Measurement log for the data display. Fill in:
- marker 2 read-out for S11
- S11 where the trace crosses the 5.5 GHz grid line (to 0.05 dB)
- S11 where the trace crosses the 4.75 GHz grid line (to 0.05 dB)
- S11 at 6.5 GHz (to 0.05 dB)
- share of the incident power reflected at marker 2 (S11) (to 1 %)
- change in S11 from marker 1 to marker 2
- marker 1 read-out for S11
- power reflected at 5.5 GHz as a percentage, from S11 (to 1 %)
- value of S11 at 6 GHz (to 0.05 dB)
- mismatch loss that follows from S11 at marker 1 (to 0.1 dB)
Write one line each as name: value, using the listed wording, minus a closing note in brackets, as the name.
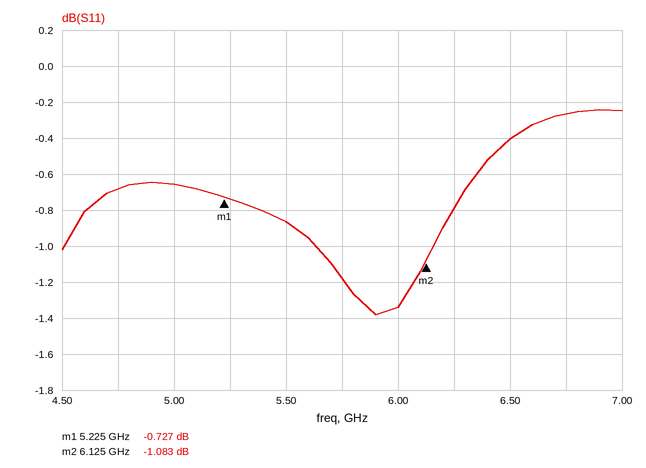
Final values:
marker 2 read-out for S11: -1.083 dB
S11 where the trace crosses the 5.5 GHz grid line: -0.85 dB
S11 where the trace crosses the 4.75 GHz grid line: -0.70 dB
S11 at 6.5 GHz: -0.40 dB
share of the incident power reflected at marker 2 (S11): 78 %
change in S11 from marker 1 to marker 2: -0.356 dB
marker 1 read-out for S11: -0.727 dB
power reflected at 5.5 GHz as a percentage, from S11: 82 %
value of S11 at 6 GHz: -1.35 dB
mismatch loss that follows from S11 at marker 1: 8.1 dB
